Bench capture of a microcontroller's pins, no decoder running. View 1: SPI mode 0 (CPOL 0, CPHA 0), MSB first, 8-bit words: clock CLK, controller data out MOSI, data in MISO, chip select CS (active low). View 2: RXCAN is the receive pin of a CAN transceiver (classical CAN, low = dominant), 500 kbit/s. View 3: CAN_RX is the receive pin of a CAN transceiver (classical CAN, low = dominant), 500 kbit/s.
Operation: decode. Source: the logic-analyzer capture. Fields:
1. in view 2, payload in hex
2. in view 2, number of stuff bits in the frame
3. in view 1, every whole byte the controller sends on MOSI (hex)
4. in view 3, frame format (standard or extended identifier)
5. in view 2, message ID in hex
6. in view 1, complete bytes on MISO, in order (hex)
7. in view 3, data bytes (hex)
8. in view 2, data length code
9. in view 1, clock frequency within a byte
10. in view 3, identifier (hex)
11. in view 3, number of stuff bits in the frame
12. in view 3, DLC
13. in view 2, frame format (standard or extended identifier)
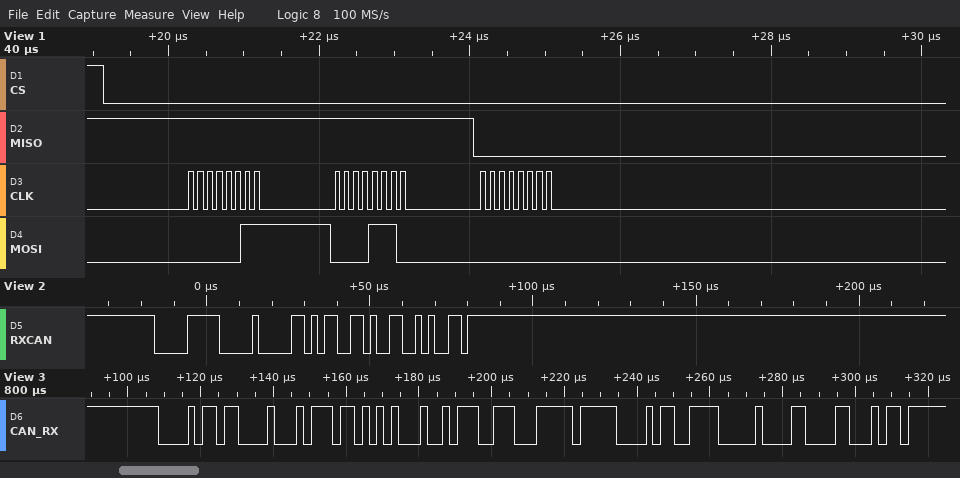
59
4
03 0E 00
standard
0x078
FF FF 00
BB 54 4B 9C 7F E2 CF 00
1
8 MHz
0x0B6
3
8
standard
